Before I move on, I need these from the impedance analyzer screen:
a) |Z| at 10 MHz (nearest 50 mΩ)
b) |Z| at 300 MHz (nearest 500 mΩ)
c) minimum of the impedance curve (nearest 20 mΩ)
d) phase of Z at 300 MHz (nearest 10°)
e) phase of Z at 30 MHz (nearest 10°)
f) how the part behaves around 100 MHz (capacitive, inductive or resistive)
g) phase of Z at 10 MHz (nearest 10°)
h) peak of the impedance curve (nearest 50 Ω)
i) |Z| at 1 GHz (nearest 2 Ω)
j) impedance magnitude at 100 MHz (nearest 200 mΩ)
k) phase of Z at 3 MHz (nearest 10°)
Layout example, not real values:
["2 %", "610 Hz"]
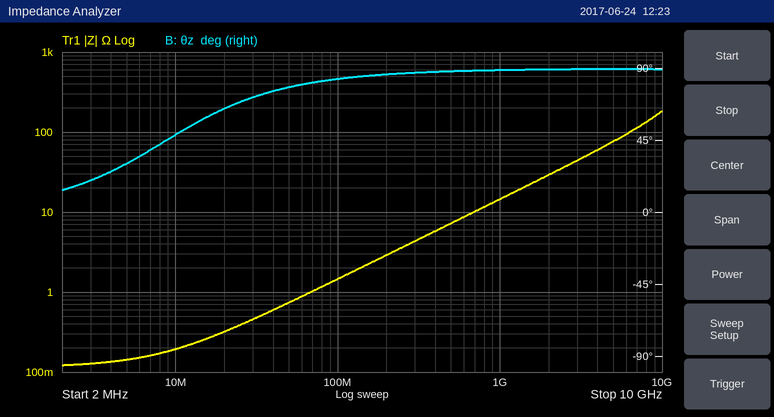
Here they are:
["200 mΩ", "4.5 Ω", "120 mΩ", "90°", "70°", "inductive", "50°", "200 Ω", "14 Ω", "1.4 Ω", "20°"]
